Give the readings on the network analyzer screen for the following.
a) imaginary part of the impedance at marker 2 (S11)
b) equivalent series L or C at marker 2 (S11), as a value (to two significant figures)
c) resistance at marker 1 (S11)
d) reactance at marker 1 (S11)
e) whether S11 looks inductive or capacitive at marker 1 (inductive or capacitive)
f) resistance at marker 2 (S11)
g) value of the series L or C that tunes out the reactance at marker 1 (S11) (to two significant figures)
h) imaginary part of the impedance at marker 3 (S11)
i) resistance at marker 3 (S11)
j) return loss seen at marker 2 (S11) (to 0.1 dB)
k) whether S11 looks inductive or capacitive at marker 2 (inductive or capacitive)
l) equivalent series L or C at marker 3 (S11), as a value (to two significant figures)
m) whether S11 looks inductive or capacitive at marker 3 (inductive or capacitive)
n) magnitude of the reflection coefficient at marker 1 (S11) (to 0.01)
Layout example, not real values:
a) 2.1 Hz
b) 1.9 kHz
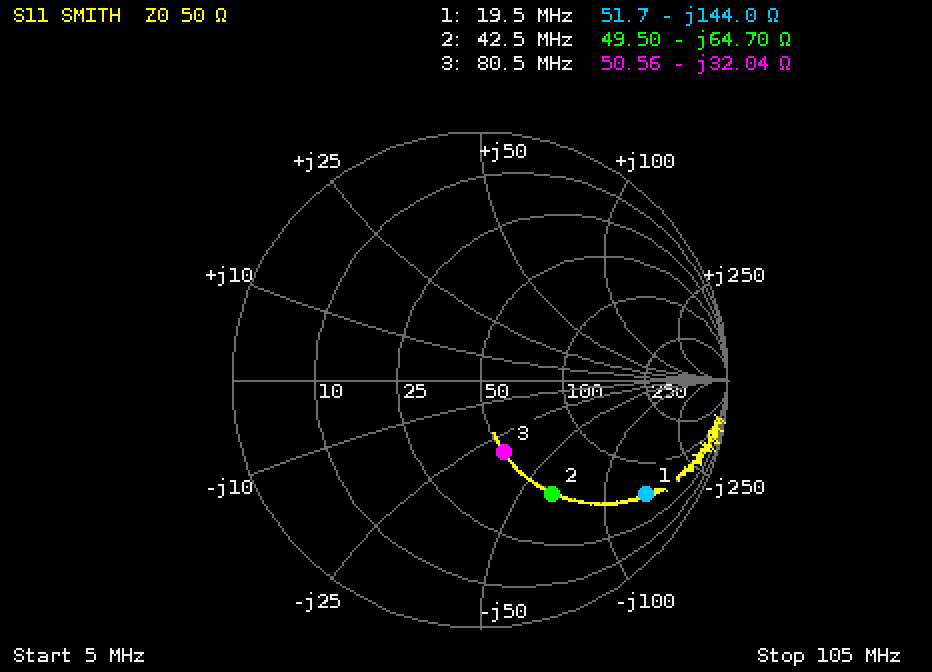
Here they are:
a) -64.70 Ω
b) 58 pF
c) 51.7 Ω
d) -144.0 Ω
e) capacitive
f) 49.50 Ω
g) 1.2 µH
h) -32.04 Ω
i) 50.56 Ω
j) 5.3 dB
k) capacitive
l) 62 pF
m) capacitive
n) 0.82
